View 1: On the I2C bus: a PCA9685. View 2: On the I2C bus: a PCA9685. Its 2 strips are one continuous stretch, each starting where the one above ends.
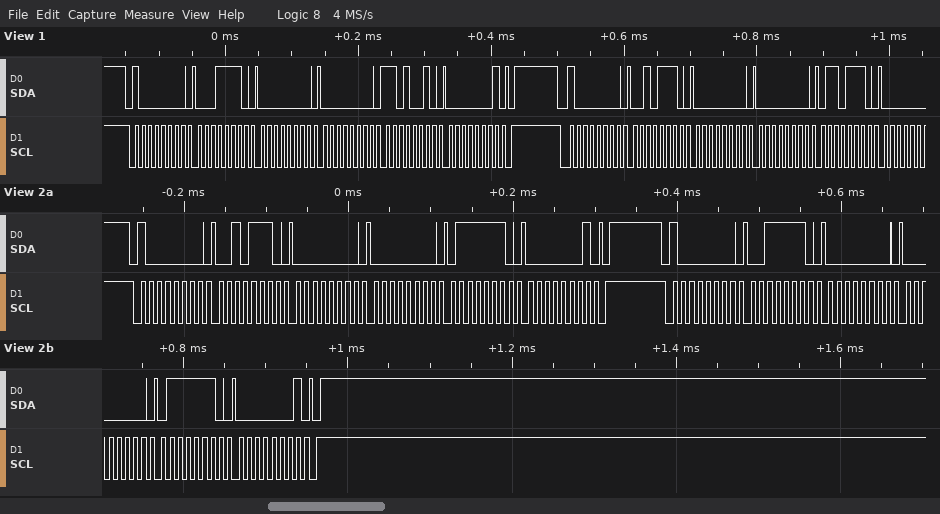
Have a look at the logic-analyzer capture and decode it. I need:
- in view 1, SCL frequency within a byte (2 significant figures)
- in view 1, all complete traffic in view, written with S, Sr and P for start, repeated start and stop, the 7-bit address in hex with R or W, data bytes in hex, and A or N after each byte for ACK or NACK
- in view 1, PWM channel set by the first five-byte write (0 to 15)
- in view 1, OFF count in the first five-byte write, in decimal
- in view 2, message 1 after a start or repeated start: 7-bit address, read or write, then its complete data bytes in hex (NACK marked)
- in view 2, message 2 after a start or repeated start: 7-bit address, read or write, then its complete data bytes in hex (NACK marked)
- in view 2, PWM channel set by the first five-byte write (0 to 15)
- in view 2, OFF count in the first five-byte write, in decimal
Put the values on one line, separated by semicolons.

100 kHz; S 40W A 1E A 00 A 00 A D2 A 01 A P S 40W A 2E A 00 A 00 A 6E A; 6; 466; 0x40 write: 2E 00 00 7E 01; 0x40 write: 3E 00 00 7E 01; 10; 382
